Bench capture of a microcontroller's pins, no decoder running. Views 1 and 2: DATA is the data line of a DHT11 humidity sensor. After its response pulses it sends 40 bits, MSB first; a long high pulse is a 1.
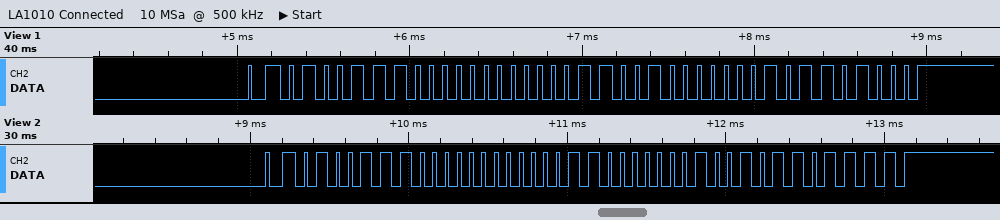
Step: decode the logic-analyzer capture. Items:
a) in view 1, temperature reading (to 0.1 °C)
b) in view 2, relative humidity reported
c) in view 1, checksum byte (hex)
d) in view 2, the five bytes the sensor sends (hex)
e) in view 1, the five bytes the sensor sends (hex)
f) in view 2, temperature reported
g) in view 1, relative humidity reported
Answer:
25.1 °C
78 %
0x68
4E 00 18 09 6F
4E 00 19 01 68
24.9 °C
78 %
